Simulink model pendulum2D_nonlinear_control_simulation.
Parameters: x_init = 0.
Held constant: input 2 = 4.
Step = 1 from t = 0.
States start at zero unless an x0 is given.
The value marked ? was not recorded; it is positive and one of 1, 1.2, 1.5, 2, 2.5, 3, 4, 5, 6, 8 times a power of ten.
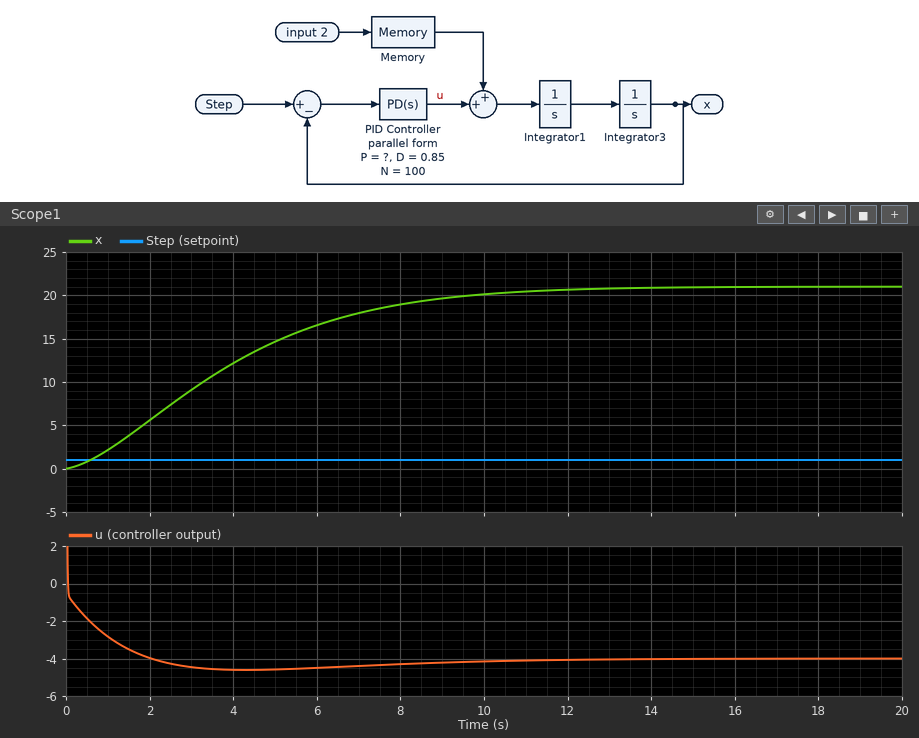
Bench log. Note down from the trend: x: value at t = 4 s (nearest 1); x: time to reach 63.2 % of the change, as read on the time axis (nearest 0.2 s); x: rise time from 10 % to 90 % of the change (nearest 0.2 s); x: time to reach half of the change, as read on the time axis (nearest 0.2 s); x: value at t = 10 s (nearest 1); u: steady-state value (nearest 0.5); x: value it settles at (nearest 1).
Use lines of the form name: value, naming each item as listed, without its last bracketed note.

x: value at t = 4 s: 12
x: time to reach 63.2 % of the change, as read on the time axis: 4.4 s
x: rise time from 10 % to 90 % of the change: 7.0 s
x: time to reach half of the change, as read on the time axis: 3.4 s
x: value at t = 10 s: 20
u: steady-state value: -4.0
x: value it settles at: 21
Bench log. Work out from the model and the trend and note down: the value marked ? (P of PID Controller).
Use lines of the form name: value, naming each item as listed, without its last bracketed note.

the value marked ?: 0.2
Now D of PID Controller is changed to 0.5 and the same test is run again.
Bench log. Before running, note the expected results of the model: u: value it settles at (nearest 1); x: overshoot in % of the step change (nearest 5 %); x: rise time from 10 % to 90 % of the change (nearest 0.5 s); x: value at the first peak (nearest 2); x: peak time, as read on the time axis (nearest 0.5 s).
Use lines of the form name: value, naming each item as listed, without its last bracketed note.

u: value it settles at: -4
x: overshoot in % of the step change: 10 %
x: rise time from 10 % to 90 % of the change: 4.0 s
x: value at the first peak: 24
x: peak time, as read on the time axis: 8.5 s
